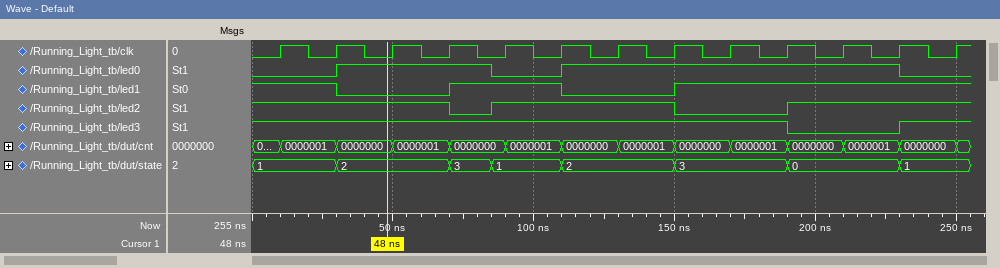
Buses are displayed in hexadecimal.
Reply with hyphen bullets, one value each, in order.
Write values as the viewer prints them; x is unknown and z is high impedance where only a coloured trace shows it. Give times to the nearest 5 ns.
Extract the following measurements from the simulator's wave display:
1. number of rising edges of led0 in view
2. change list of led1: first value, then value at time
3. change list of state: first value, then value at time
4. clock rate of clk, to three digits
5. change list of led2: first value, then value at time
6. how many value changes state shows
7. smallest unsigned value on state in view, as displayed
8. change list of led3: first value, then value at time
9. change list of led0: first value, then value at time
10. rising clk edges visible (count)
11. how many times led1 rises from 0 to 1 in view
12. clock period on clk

- 2
- 1, 0 at 30 ns, 1 at 70 ns, 0 at 110 ns, 1 at 150 ns
- 1, 2 at 30 ns, 3 at 70 ns, 1 at 85 ns, 2 at 110 ns, 3 at 150 ns, 0 at 190 ns, 1 at 230 ns
- 50.0 MHz
- 1, 0 at 70 ns, 1 at 85 ns, 0 at 150 ns, 1 at 190 ns
- 7
- 0
- 1, 0 at 190 ns, 1 at 230 ns
- 0, 1 at 30 ns, 0 at 85 ns, 1 at 110 ns, 0 at 230 ns
- 13
- 2
- 20 ns
